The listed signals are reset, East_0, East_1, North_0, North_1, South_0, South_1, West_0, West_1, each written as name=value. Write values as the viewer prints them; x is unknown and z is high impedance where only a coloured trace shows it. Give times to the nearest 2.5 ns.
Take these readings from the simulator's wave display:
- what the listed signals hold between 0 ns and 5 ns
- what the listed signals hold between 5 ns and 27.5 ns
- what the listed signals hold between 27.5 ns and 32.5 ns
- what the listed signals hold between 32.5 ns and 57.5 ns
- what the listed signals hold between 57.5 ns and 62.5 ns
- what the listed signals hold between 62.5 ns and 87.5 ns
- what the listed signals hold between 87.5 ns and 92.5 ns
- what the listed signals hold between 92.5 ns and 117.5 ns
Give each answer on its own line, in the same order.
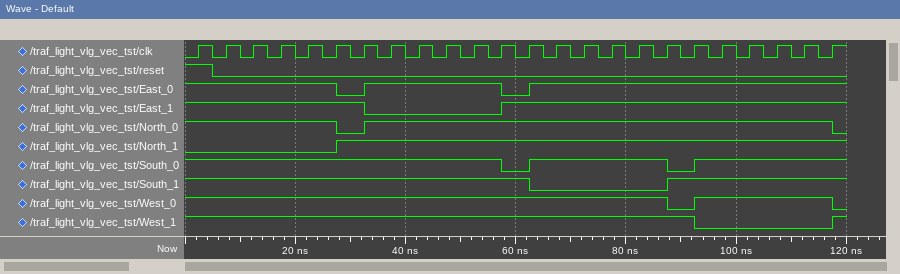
reset=1, East_0=1, East_1=1, North_0=1, North_1=0, South_0=1, South_1=1, West_0=1, West_1=1
reset=0, East_0=1, East_1=1, North_0=1, North_1=0, South_0=1, South_1=1, West_0=1, West_1=1
reset=0, East_0=0, East_1=1, North_0=0, North_1=1, South_0=1, South_1=1, West_0=1, West_1=1
reset=0, East_0=1, East_1=0, North_0=1, North_1=1, South_0=1, South_1=1, West_0=1, West_1=1
reset=0, East_0=0, East_1=1, North_0=1, North_1=1, South_0=0, South_1=1, West_0=1, West_1=1
reset=0, East_0=1, East_1=1, North_0=1, North_1=1, South_0=1, South_1=0, West_0=1, West_1=1
reset=0, East_0=1, East_1=1, North_0=1, North_1=1, South_0=0, South_1=1, West_0=0, West_1=1
reset=0, East_0=1, East_1=1, North_0=1, North_1=1, South_0=1, South_1=1, West_0=1, West_1=0
